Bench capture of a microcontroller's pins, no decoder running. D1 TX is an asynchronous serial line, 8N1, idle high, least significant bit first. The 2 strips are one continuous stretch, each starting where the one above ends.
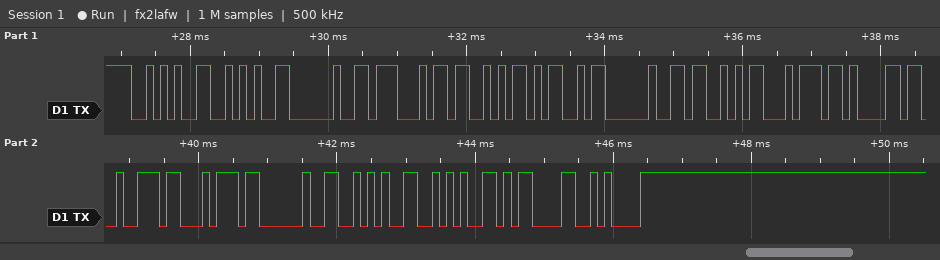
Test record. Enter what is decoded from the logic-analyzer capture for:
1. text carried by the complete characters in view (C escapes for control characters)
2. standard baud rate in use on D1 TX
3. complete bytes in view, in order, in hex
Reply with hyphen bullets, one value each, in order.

- "** GSM Start **\r\n"
- 9600 baud
- 0x2A 0x2A 0x20 0x47 0x53 0x4D 0x20 0x53 0x74 0x61 0x72 0x74 0x20 0x2A 0x2A 0x0D 0x0A
